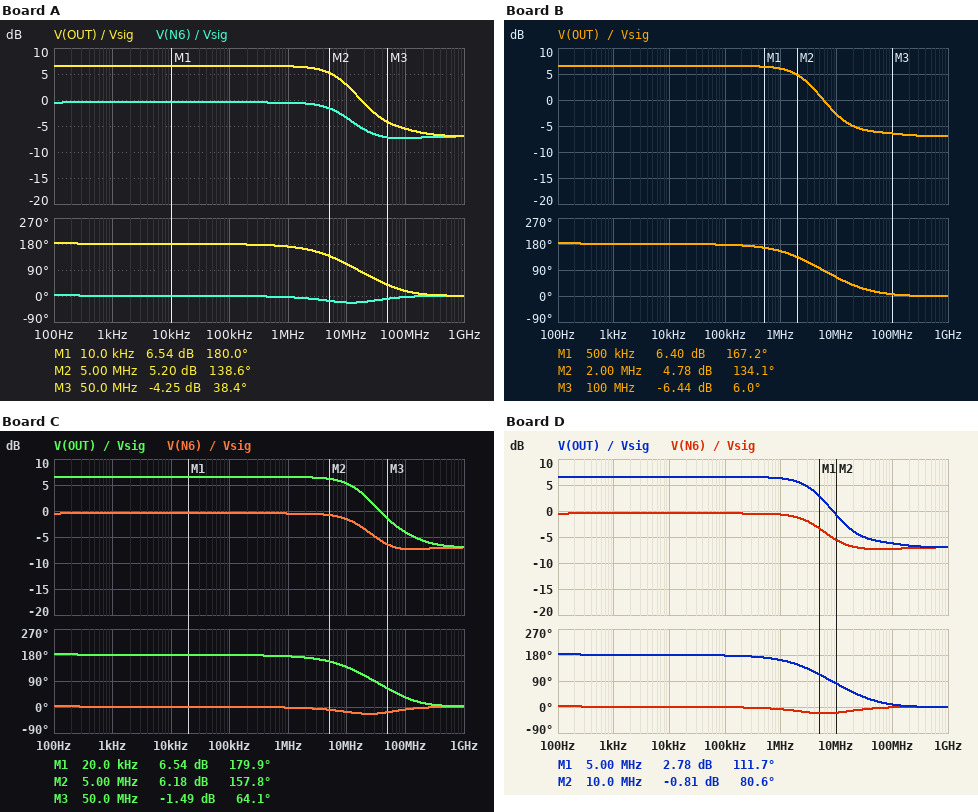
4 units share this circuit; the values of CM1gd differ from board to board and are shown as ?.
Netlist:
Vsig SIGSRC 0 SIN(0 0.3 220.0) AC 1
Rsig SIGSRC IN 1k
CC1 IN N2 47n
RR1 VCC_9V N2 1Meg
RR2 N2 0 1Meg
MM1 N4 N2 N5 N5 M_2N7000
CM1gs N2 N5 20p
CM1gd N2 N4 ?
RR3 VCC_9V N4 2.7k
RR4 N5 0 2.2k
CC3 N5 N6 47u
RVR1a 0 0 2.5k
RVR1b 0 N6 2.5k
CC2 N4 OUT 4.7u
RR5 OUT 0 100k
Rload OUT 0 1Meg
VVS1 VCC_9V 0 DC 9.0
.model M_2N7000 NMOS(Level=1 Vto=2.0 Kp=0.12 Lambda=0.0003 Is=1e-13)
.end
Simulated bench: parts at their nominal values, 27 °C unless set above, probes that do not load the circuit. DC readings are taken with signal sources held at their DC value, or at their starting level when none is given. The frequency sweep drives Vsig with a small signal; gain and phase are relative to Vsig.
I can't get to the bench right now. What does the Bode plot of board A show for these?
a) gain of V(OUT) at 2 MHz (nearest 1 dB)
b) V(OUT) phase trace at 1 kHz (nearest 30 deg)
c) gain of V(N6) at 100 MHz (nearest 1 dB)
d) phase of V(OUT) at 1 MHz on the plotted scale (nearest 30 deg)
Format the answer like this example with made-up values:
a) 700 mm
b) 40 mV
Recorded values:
a) 6 dB
b) 180 deg
c) -7 dB
d) 180 deg
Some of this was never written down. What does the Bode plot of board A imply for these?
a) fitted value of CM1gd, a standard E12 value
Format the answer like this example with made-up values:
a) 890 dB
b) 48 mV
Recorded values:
a) 3.3 pF
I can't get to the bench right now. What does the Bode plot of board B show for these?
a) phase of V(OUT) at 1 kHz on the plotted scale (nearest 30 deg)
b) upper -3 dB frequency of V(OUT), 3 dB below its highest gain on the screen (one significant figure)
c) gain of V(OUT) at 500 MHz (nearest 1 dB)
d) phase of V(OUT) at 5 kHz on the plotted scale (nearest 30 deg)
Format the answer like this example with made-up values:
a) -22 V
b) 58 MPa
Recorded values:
a) 180 deg
b) 3 MHz
c) -7 dB
d) 180 deg
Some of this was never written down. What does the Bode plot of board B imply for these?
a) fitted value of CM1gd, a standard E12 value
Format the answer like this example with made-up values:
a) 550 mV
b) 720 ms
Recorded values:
a) 10 pF
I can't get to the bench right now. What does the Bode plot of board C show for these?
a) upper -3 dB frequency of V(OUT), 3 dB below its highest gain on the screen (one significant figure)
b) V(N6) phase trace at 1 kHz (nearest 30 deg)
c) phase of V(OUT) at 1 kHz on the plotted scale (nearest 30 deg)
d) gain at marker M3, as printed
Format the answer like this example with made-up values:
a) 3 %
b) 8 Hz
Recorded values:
a) 20 MHz
b) 0 deg
c) 180 deg
d) -1.49 dB
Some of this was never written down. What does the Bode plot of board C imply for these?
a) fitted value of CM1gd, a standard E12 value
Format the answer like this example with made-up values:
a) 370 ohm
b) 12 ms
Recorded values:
a) 1.5 pF
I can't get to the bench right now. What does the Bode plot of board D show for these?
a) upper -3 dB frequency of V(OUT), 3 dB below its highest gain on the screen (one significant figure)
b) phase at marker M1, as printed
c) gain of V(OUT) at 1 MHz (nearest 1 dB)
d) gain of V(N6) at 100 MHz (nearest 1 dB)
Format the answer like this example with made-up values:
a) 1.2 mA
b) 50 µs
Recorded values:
a) 4 MHz
b) 111.7 deg
c) 6 dB
d) -7 dB
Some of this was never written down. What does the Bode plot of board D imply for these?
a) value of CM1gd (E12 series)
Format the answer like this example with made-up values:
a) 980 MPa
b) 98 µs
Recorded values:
a) 6.8 pF
